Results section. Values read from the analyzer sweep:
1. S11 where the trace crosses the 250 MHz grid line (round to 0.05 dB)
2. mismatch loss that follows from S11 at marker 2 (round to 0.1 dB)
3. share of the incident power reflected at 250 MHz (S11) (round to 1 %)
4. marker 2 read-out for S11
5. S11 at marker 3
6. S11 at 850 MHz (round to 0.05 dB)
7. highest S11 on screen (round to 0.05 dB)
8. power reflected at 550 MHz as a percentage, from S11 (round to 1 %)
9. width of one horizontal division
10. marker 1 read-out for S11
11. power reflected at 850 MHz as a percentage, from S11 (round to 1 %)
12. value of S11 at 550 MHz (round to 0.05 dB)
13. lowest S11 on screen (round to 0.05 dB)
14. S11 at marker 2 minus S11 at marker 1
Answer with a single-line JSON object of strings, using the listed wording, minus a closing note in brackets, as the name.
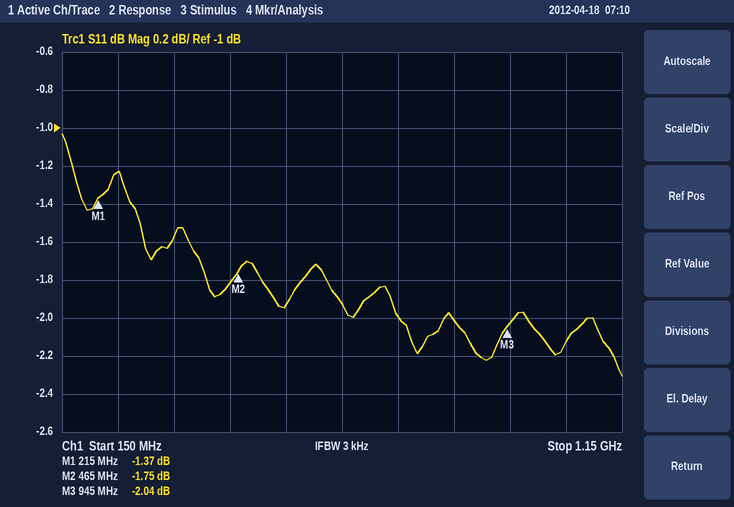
{"S11 where the trace crosses the 250 MHz grid line": "-1.25 dB", "mismatch loss that follows from S11 at marker 2": "4.8 dB", "share of the incident power reflected at 250 MHz (S11)": "75 %", "marker 2 read-out for S11": "-1.75 dB", "S11 at marker 3": "-2.04 dB", "S11 at 850 MHz": "-2.00 dB", "highest S11 on screen": "-1.05 dB", "power reflected at 550 MHz as a percentage, from S11": "64 %", "width of one horizontal division": "100 MHz", "marker 1 read-out for S11": "-1.37 dB", "power reflected at 850 MHz as a percentage, from S11": "63 %", "value of S11 at 550 MHz": "-1.95 dB", "lowest S11 on screen": "-2.30 dB", "S11 at marker 2 minus S11 at marker 1": "-0.38 dB"}
